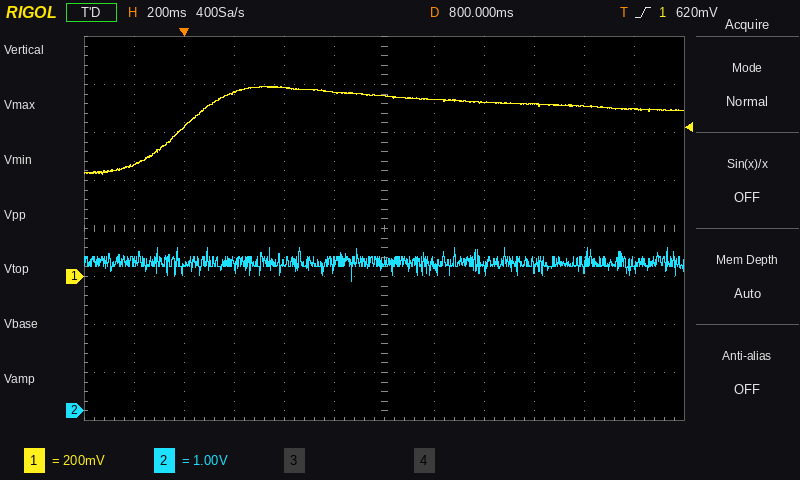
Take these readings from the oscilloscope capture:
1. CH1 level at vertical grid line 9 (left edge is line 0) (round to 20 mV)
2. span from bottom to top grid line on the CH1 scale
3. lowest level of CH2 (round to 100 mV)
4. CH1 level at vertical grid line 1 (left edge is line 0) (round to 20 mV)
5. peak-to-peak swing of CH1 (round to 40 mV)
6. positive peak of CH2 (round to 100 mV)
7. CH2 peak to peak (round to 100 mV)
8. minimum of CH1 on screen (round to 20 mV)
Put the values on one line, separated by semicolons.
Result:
720 mV; 1.6 V; 2.7 V; 460 mV; 360 mV; 3.4 V; 700 mV; 420 mV
